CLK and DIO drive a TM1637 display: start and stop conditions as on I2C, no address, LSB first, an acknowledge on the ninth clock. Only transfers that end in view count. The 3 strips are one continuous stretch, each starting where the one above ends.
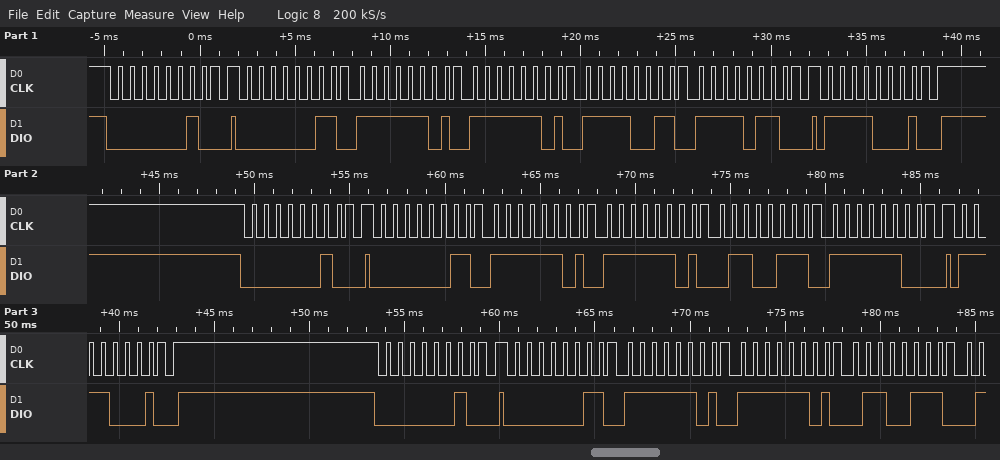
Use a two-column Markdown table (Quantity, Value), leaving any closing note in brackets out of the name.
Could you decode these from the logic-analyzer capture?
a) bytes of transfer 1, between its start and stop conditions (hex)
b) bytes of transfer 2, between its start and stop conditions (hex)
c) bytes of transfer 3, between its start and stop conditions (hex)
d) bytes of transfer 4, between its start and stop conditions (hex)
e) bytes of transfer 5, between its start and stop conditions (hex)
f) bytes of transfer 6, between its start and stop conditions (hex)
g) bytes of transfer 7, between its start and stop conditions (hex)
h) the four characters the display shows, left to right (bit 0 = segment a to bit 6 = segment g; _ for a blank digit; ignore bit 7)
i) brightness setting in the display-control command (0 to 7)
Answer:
| Quantity | Value |
|---|---|
| bytes of transfer 1, between its start and stop conditions | 40 |
| bytes of transfer 2, between its start and stop conditions | C0 BF BF CF 6F |
| bytes of transfer 3, between its start and stop conditions | 8F |
| bytes of transfer 4, between its start and stop conditions | 40 |
| bytes of transfer 5, between its start and stop conditions | C0 BF BF E6 3F |
| bytes of transfer 6, between its start and stop conditions | 8F |
| bytes of transfer 7, between its start and stop conditions | 40 |
| the four characters the display shows, left to right | 0040 |
| brightness setting in the display-control command | 7 |
